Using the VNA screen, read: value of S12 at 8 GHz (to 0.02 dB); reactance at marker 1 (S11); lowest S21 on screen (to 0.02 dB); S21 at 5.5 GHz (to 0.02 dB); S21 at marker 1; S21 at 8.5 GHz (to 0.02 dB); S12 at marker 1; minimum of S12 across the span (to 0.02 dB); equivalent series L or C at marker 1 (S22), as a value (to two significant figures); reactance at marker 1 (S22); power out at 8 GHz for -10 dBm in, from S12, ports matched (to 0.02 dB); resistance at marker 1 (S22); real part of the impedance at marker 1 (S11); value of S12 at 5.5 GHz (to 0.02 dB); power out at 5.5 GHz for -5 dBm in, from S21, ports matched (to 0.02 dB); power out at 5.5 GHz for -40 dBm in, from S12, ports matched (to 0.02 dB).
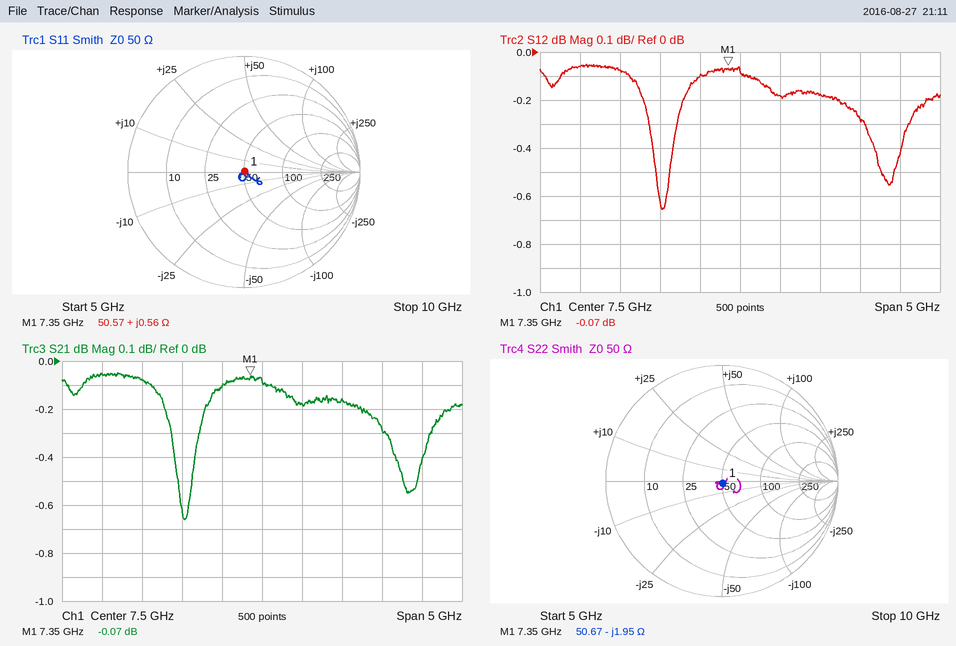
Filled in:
-0.18 dB
+0.56 Ω
-0.66 dB
-0.06 dB
-0.07 dB
-0.16 dB
-0.07 dB
-0.66 dB
11 pF
-1.95 Ω
-10.18 dBm
50.67 Ω
50.57 Ω
-0.06 dB
-5.06 dBm
-40.06 dBm
